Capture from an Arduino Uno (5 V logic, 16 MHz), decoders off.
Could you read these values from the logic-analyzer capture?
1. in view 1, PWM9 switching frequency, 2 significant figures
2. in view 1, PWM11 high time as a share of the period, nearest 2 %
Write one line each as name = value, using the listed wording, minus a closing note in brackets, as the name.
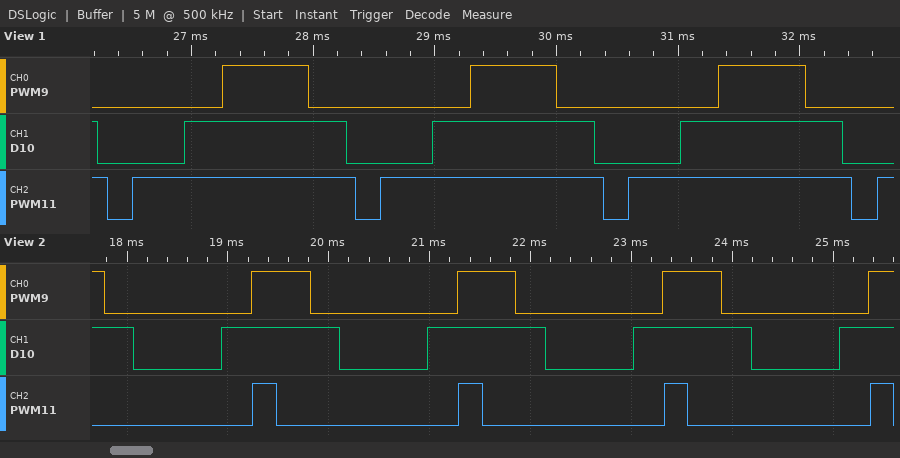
in view 1, PWM9 switching frequency, 2 significant figures = 490 Hz
in view 1, PWM11 high time as a share of the period, nearest 2 % = 90 %
